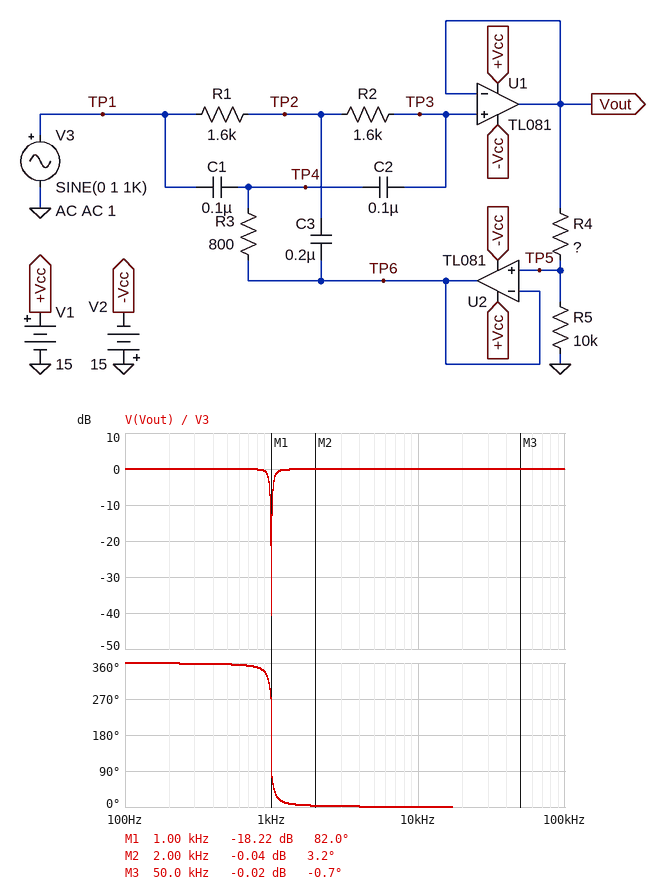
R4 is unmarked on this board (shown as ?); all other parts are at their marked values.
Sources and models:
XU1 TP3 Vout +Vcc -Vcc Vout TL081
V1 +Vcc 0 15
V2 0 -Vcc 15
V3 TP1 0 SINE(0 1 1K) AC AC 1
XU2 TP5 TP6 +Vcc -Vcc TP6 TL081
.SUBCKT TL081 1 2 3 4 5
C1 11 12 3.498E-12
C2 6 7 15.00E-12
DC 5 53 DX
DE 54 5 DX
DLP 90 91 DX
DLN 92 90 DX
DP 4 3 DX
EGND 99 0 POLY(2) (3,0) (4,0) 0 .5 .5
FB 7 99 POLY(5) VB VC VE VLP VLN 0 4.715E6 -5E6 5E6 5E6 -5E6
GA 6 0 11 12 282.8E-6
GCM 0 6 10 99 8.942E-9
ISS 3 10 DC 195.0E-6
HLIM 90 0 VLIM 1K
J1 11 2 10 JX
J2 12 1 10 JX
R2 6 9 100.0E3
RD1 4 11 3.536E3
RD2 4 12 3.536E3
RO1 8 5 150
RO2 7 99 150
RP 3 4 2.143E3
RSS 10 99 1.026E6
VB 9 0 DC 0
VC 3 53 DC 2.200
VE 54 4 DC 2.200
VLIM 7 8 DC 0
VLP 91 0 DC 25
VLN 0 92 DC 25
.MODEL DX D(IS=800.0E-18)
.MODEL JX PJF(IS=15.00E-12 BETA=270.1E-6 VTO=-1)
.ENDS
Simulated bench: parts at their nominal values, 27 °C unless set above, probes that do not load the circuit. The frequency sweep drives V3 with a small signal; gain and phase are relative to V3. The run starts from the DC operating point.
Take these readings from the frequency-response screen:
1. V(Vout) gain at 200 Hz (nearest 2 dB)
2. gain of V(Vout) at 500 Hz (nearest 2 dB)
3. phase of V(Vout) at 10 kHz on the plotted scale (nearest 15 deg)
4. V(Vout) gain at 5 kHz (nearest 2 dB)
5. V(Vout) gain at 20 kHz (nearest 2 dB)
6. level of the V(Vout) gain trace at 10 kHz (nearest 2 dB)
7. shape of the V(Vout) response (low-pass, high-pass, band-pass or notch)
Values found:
0 dB
0 dB
0 deg
0 dB
0 dB
0 dB
notch
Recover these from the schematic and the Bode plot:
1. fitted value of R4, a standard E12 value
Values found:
220 Ω
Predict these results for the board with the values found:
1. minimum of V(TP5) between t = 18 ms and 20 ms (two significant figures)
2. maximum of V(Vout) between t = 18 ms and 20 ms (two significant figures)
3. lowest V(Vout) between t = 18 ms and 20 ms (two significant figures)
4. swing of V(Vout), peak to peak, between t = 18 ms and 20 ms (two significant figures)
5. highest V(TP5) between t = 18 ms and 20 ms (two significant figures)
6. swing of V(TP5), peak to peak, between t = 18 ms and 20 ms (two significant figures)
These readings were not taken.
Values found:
-120 mV
120 mV
-120 mV
240 mV
120 mV
230 mV
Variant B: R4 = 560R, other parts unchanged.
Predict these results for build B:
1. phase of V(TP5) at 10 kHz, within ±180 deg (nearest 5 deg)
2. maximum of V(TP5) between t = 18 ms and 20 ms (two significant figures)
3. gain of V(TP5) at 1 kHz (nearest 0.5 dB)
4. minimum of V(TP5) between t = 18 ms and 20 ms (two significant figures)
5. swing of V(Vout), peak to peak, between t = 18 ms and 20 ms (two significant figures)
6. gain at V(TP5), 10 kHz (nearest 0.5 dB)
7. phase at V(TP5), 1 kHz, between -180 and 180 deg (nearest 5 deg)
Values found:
0 deg
48 mV
-26.5 dB
-48 mV
100 mV
-0.5 dB
85 deg
